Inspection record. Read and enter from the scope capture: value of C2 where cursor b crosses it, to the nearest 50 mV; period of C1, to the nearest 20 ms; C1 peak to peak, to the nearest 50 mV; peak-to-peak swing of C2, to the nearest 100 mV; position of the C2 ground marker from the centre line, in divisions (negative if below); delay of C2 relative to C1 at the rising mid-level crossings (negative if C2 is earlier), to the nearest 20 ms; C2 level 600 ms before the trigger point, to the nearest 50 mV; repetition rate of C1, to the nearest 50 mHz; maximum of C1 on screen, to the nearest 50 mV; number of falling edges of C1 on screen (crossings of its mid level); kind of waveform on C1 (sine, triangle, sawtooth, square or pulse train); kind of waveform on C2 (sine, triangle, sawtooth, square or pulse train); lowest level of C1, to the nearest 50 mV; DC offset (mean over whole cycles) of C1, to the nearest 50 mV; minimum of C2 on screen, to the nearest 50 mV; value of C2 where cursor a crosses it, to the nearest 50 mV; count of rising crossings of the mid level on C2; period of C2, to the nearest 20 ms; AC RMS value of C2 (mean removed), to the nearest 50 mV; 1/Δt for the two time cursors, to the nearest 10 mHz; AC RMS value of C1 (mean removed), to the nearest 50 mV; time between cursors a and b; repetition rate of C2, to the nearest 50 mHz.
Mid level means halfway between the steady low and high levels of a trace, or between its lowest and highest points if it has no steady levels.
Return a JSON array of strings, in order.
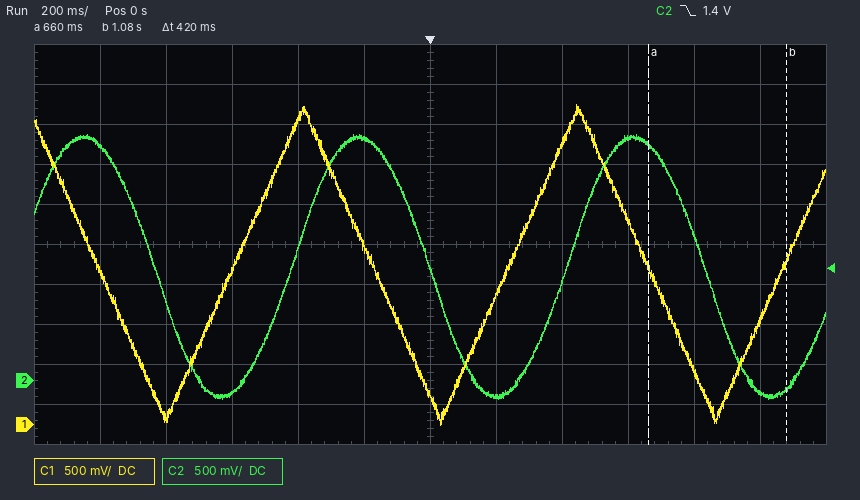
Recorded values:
["-100 mV", "840 ms", "4.00 V", "3.30 V", "-3.4 div", "+180 ms", "-150 mV", "1.20 Hz", "4.00 V", "3", "triangle", "sine", "0 mV", "2.00 V", "-250 mV", "2.95 V", "2", "840 ms", "1.15 V", "2.38 Hz", "1.15 V", "420 ms", "1.20 Hz"]
